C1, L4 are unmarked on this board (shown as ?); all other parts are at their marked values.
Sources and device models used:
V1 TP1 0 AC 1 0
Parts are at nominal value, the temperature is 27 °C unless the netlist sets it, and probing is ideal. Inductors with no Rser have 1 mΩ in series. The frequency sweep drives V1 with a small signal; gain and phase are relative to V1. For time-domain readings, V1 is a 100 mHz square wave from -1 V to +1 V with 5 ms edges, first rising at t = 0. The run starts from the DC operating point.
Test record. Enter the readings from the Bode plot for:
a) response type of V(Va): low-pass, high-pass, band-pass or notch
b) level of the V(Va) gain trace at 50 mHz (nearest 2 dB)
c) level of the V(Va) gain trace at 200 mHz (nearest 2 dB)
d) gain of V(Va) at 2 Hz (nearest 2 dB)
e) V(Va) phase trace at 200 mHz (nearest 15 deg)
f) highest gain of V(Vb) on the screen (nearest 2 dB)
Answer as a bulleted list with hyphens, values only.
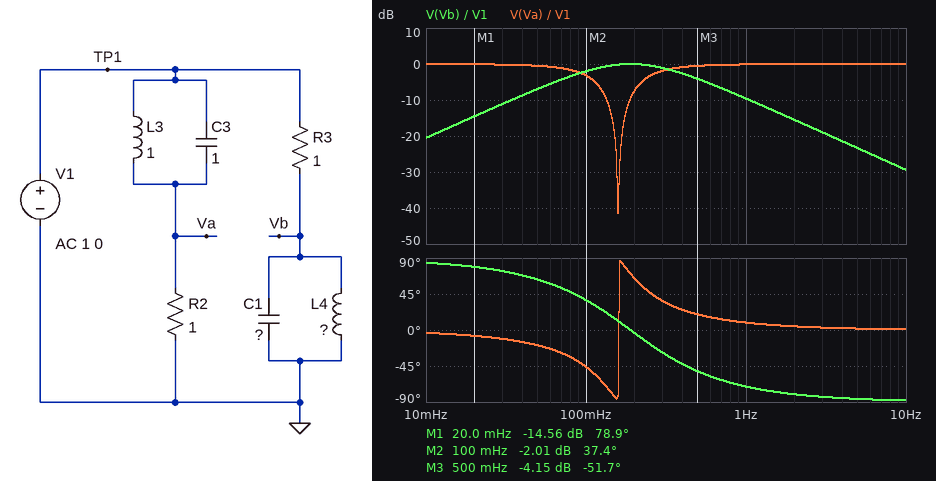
- notch
- 0 dB
- -8 dB
- 0 dB
- 60 deg
- 0 dB
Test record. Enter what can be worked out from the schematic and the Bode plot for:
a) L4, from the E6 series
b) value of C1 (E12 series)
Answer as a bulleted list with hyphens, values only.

- 1.5 H
- 470 mF
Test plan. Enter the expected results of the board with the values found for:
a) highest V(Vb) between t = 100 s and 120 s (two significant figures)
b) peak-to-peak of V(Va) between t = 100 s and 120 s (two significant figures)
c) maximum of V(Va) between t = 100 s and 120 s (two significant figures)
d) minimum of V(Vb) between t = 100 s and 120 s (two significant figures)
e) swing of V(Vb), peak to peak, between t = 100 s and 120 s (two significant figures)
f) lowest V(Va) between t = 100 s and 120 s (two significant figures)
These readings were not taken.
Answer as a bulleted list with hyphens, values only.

- 1.4 V
- 2.4 V
- 1.2 V
- -1.4 V
- 2.8 V
- -1.2 V
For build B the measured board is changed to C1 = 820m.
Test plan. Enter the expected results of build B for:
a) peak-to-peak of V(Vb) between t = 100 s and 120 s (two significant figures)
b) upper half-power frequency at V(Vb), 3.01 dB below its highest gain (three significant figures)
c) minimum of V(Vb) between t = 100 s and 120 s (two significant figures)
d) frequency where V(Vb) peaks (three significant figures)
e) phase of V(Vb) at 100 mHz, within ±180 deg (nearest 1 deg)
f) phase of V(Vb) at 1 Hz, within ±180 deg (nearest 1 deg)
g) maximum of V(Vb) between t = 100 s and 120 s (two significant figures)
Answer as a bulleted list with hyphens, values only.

- 2.7 V
- 270 mHz
- -1.3 V
- 144 mHz
- 29 deg
- -79 deg
- 1.3 V
